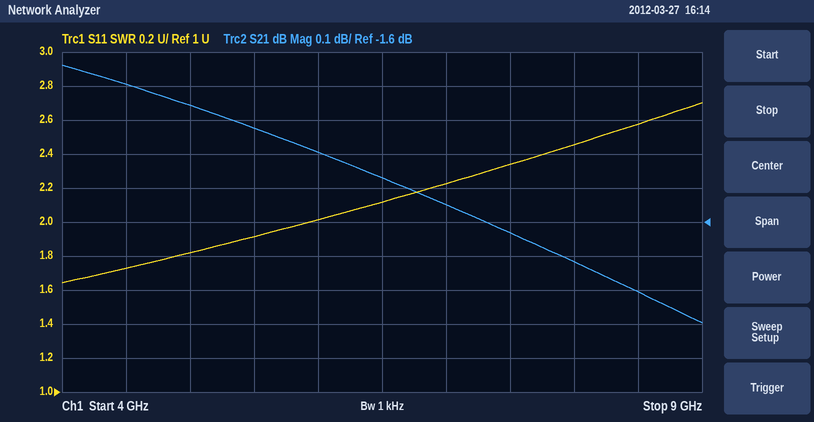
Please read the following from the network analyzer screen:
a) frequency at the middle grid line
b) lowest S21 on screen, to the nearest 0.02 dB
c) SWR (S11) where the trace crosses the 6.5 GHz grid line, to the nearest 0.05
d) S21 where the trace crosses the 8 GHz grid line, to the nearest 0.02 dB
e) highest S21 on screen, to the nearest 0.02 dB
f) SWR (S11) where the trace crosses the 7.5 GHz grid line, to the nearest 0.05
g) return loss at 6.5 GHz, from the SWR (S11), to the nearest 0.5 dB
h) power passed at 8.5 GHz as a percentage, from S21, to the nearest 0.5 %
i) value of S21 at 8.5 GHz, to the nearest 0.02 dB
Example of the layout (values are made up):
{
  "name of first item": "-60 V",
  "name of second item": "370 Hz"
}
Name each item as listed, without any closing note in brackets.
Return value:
{
  "frequency at the middle grid line": "6.5 GHz",
  "lowest S21 on screen, to the nearest 0.02 dB": "-1.90 dB",
  "SWR (S11) where the trace crosses the 6.5 GHz grid line, to the nearest 0.05": "2.10",
  "S21 where the trace crosses the 8 GHz grid line, to the nearest 0.02 dB": "-1.72 dB",
  "highest S21 on screen, to the nearest 0.02 dB": "-1.14 dB",
  "SWR (S11) where the trace crosses the 7.5 GHz grid line, to the nearest 0.05": "2.35",
  "return loss at 6.5 GHz, from the SWR (S11), to the nearest 0.5 dB": "9.0 dB",
  "power passed at 8.5 GHz as a percentage, from S21, to the nearest 0.5 %": "66.0 %",
  "value of S21 at 8.5 GHz, to the nearest 0.02 dB": "-1.80 dB"
}
